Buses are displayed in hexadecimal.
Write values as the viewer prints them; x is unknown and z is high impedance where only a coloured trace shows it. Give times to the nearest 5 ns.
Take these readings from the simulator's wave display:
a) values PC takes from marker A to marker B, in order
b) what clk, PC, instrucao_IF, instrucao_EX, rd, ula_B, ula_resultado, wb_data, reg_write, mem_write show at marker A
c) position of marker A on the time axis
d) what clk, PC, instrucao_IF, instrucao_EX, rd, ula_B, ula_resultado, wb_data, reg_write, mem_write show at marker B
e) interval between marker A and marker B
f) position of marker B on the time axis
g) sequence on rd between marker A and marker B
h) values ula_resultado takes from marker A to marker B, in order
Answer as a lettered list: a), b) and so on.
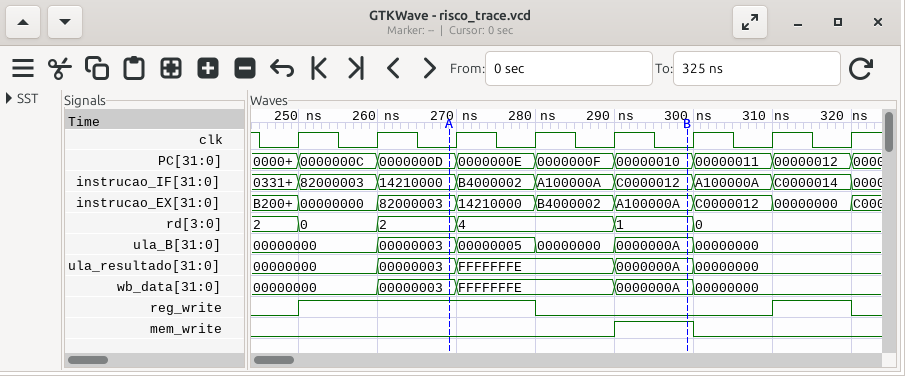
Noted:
a) 0000000D, 0000000E, 0000000F, 00000010
b) clk=0, PC=0000000D, instrucao_IF=14210000, instrucao_EX=82000003, rd=2, ula_B=00000003, ula_resultado=00000003, wb_data=00000003, reg_write=1, mem_write=0
c) 270 ns
d) clk=0, PC=00000010, instrucao_IF=C0000012, instrucao_EX=A100000A, rd=1, ula_B=0000000A, ula_resultado=0000000A, wb_data=0000000A, reg_write=0, mem_write=1
e) 30 ns
f) 300 ns
g) 2, 4, 1
h) 00000003, FFFFFFFE, 0000000A
